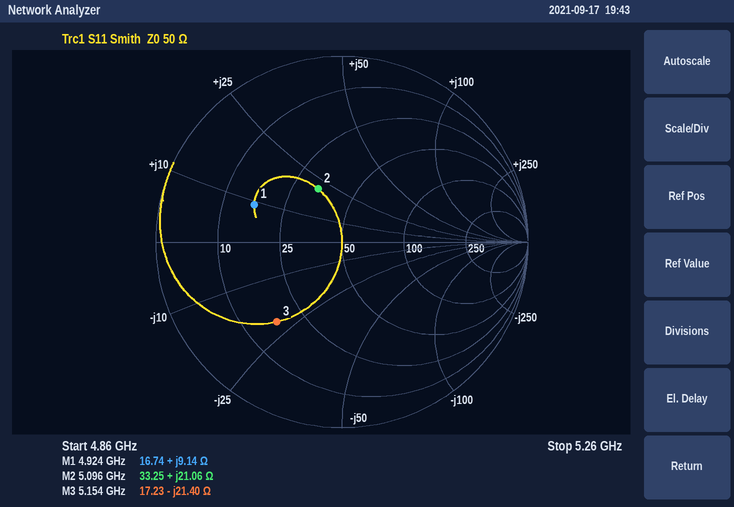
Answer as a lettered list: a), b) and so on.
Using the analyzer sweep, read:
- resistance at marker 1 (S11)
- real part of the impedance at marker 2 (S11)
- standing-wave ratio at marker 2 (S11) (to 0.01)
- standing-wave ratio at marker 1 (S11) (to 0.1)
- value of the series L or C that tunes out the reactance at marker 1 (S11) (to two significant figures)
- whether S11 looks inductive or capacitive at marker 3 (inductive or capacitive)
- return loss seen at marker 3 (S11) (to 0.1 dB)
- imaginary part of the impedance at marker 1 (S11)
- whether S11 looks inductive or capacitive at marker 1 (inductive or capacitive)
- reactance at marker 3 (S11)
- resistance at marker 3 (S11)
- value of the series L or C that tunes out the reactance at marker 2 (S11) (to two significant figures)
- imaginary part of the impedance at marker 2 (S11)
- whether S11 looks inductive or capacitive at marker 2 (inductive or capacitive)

a) 16.74 Ω
b) 33.25 Ω
c) 1.91
d) 3.1
e) 3.5 pF
f) capacitive
g) 5.1 dB
h) +9.14 Ω
i) inductive
j) -21.40 Ω
k) 17.23 Ω
l) 1.5 pF
m) +21.06 Ω
n) inductive
